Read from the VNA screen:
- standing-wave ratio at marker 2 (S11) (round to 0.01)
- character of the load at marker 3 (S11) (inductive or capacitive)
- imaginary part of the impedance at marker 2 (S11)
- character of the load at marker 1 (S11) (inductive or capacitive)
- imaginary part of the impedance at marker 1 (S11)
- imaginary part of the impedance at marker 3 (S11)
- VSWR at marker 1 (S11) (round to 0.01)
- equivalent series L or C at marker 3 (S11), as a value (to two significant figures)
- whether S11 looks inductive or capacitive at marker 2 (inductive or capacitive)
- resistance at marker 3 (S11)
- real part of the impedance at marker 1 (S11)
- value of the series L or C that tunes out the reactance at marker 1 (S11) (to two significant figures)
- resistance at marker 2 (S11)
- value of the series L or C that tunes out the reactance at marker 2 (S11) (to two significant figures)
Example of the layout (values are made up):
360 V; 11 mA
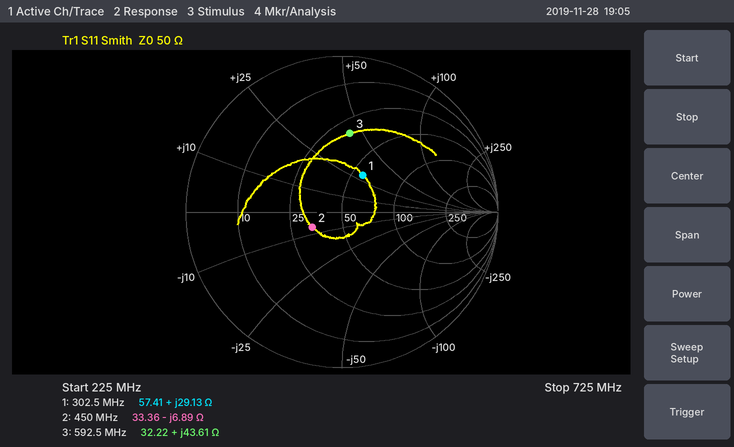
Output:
1.55; inductive; -6.89 Ω; inductive; +29.13 Ω; +43.61 Ω; 1.74; 12 nH; capacitive; 32.22 Ω; 57.41 Ω; 18 pF; 33.36 Ω; 2.4 nH
